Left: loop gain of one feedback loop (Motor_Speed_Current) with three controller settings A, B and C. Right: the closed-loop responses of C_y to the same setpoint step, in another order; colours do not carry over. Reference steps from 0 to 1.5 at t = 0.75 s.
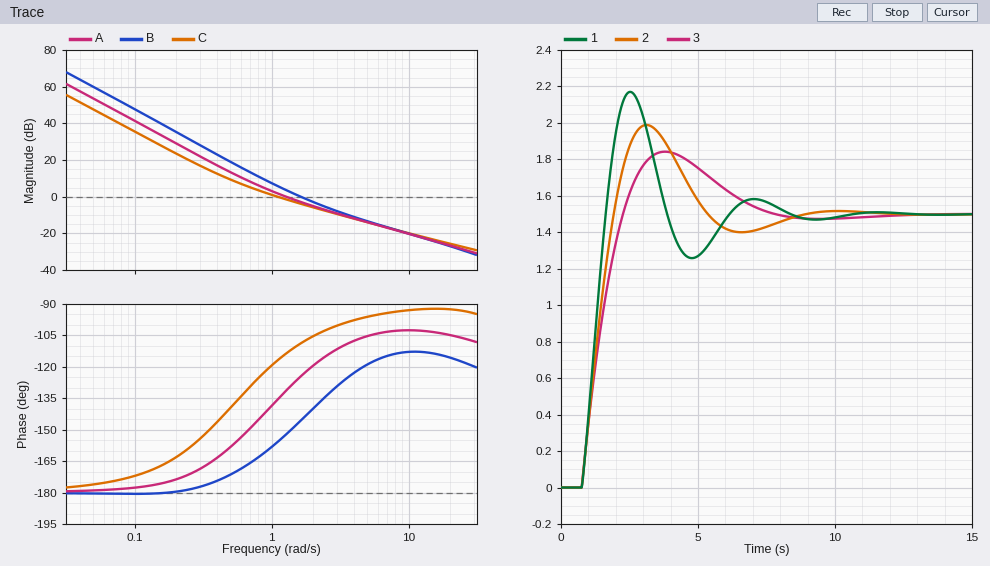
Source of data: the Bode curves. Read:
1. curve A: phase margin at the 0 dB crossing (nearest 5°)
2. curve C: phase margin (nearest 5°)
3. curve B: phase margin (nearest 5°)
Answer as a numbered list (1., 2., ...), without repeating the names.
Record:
1. 50°
2. 65°
3. 35°
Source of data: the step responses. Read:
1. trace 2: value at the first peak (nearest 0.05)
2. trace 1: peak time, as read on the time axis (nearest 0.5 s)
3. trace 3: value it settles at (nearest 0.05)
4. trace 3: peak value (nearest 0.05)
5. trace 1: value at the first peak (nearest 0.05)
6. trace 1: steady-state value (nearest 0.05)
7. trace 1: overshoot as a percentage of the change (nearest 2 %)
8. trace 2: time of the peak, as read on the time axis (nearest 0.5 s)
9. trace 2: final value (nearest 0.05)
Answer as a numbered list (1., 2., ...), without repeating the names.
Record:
1. 2.00
2. 2.5 s
3. 1.50
4. 1.85
5. 2.15
6. 1.50
7. 44 %
8. 3.0 s
9. 1.50
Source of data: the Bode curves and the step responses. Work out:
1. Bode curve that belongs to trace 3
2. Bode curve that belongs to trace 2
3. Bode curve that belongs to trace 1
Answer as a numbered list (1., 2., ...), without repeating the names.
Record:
1. C
2. A
3. B
